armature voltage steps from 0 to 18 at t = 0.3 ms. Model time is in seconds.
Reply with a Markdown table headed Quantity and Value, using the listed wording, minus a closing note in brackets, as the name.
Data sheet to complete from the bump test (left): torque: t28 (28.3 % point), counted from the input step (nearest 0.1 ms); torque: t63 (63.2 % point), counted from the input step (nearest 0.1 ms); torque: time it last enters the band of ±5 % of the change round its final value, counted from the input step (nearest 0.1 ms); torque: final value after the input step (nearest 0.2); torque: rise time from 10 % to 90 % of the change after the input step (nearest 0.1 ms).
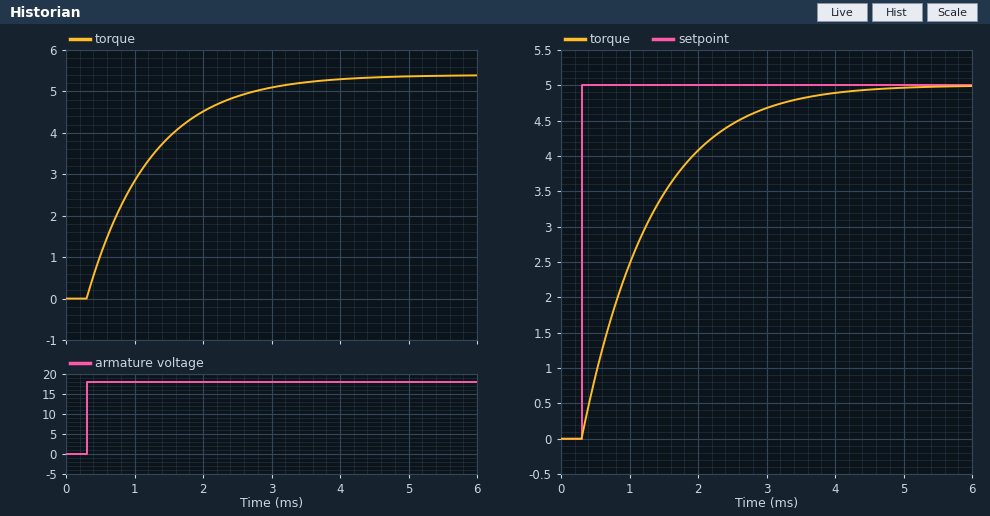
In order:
| Quantity | Value |
|---|---|
| torque: t28 (28.3 % point), counted from the input step | 0.3 ms |
| torque: t63 (63.2 % point), counted from the input step | 0.9 ms |
| torque: time it last enters the band of ±5 % of the change round its final value, counted from the input step | 2.8 ms |
| torque: final value after the input step | 5.4 |
| torque: rise time from 10 % to 90 % of the change after the input step | 2.1 ms |
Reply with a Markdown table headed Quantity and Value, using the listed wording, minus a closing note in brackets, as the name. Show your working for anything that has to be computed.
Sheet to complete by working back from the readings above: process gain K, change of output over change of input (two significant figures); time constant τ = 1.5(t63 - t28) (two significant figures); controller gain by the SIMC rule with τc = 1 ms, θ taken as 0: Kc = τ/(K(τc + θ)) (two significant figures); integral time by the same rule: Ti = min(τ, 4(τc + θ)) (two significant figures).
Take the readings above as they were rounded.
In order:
| Quantity | Value |
|---|---|
| process gain K, change of output over change of input | (5.4 - 0) / 18 = 0.30 |
| time constant τ = 1.5(t63 - t28) | 1.5 × (0.9 - 0.3) = 0.90 ms |
| controller gain by the SIMC rule with τc = 1 ms, θ taken as 0: Kc = τ/(K(τc + θ)) | 0.9 / (0.3 × (1 + 0)) = 3.0 |
| integral time by the same rule: Ti = min(τ, 4(τc + θ)) | min(0.9, 4 × (1 + 0)) = 0.90 ms |
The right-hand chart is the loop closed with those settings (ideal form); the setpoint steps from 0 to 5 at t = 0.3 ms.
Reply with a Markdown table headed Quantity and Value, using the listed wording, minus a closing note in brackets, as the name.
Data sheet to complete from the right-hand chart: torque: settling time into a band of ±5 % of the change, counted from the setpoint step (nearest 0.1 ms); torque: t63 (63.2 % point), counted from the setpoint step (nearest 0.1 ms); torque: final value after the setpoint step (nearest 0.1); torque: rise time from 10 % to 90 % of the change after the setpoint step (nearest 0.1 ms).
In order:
| Quantity | Value |
|---|---|
| torque: settling time into a band of ±5 % of the change, counted from the setpoint step | 2.9 ms |
| torque: t63 (63.2 % point), counted from the setpoint step | 1.0 ms |
| torque: final value after the setpoint step | 5.0 |
| torque: rise time from 10 % to 90 % of the change after the setpoint step | 2.2 ms |
